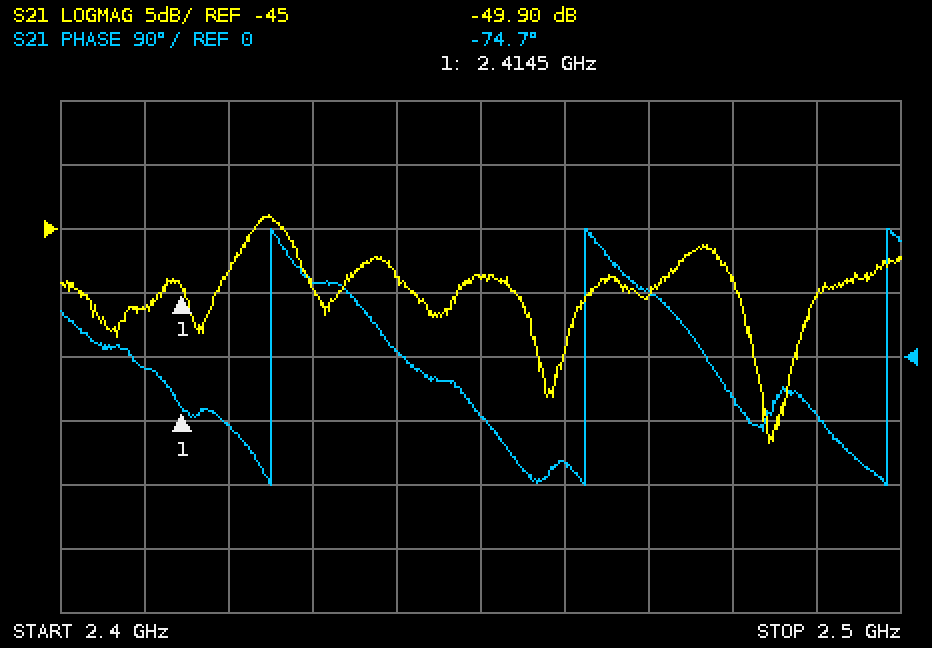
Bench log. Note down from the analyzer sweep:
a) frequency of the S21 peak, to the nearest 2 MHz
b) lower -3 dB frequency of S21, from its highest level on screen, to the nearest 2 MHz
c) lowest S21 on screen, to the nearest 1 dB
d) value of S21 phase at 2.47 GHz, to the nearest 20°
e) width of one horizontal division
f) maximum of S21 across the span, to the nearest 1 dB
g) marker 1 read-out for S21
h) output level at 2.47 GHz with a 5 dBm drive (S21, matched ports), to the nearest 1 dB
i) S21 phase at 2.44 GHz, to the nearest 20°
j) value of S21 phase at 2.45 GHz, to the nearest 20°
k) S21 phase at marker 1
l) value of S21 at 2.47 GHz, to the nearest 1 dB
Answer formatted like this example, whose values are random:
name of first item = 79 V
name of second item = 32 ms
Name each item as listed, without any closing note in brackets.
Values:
frequency of the S21 peak, to the nearest 2 MHz = 2.424 GHz
lower -3 dB frequency of S21, from its highest level on screen, to the nearest 2 MHz = 2.422 GHz
lowest S21 on screen, to the nearest 1 dB = -62 dB
value of S21 phase at 2.47 GHz, to the nearest 20° = 100°
width of one horizontal division = 10 MHz
maximum of S21 across the span, to the nearest 1 dB = -44 dB
marker 1 read-out for S21 = -49.90 dB
output level at 2.47 GHz with a 5 dBm drive (S21, matched ports), to the nearest 1 dB = -45 dBm
S21 phase at 2.44 GHz, to the nearest 20° = 0°
value of S21 phase at 2.45 GHz, to the nearest 20° = -80°
S21 phase at marker 1 = -74.7°
value of S21 at 2.47 GHz, to the nearest 1 dB = -50 dB
